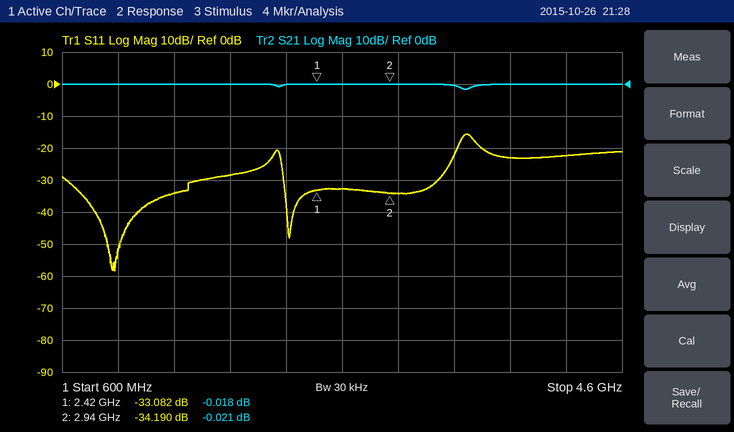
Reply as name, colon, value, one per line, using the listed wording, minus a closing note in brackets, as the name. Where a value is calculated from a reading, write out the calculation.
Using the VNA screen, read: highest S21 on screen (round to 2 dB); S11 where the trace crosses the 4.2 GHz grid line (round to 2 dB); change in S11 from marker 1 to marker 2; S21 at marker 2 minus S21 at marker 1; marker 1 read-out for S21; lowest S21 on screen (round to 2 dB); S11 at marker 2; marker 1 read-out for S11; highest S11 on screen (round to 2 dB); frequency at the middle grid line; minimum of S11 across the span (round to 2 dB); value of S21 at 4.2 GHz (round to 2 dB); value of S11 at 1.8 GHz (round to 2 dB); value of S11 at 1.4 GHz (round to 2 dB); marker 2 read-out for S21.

highest S21 on screen: 0 dB
S11 where the trace crosses the 4.2 GHz grid line: -22 dB
change in S11 from marker 1 to marker 2: -34.19 − (-33.082) = -1.108 dB
S21 at marker 2 minus S21 at marker 1: -0.021 − (-0.018) = -0.003 dB
marker 1 read-out for S21: -0.018 dB
lowest S21 on screen: -2 dB
S11 at marker 2: -34.190 dB
marker 1 read-out for S11: -33.082 dB
highest S11 on screen: -16 dB
frequency at the middle grid line: 2.6 GHz
minimum of S11 across the span: -58 dB
value of S21 at 4.2 GHz: 0 dB
value of S11 at 1.8 GHz: -28 dB
value of S11 at 1.4 GHz: -34 dB
marker 2 read-out for S21: -0.021 dB
